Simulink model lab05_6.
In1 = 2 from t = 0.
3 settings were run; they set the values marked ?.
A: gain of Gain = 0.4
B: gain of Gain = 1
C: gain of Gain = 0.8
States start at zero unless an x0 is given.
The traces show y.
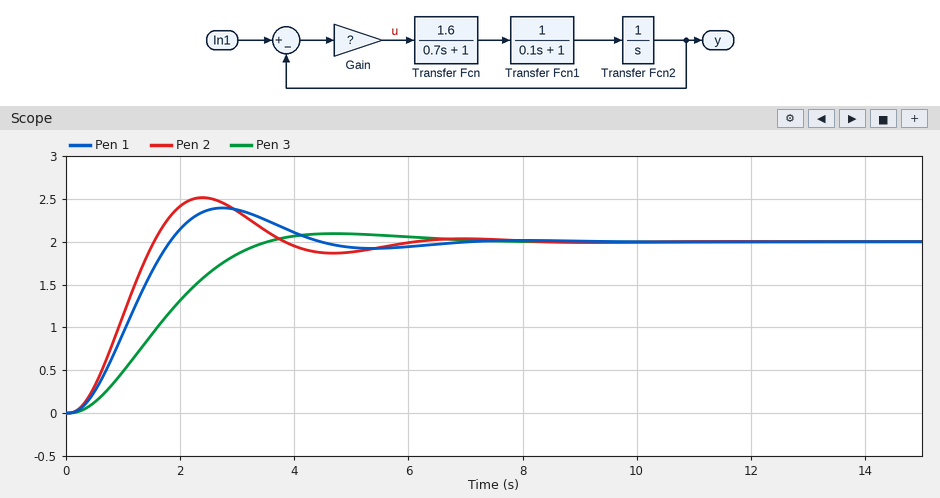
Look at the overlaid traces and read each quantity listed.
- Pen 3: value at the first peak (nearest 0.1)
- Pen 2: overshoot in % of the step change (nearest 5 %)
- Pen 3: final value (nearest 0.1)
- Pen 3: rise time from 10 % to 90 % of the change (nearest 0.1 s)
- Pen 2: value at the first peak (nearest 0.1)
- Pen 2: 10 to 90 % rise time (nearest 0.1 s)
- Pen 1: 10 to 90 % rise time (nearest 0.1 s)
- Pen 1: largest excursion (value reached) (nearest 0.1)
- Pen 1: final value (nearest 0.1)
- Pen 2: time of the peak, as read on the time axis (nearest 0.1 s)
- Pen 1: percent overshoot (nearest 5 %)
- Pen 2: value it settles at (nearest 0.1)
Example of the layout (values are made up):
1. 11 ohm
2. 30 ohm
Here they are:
1. 2.1
2. 25 %
3. 2.0
4. 2.2 s
5. 2.5
6. 1.0 s
7. 1.2 s
8. 2.4
9. 2.0
10. 2.4 s
11. 20 %
12. 2.0
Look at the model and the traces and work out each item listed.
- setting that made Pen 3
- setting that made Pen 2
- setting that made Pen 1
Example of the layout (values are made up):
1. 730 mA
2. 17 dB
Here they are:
1. A
2. B
3. C
